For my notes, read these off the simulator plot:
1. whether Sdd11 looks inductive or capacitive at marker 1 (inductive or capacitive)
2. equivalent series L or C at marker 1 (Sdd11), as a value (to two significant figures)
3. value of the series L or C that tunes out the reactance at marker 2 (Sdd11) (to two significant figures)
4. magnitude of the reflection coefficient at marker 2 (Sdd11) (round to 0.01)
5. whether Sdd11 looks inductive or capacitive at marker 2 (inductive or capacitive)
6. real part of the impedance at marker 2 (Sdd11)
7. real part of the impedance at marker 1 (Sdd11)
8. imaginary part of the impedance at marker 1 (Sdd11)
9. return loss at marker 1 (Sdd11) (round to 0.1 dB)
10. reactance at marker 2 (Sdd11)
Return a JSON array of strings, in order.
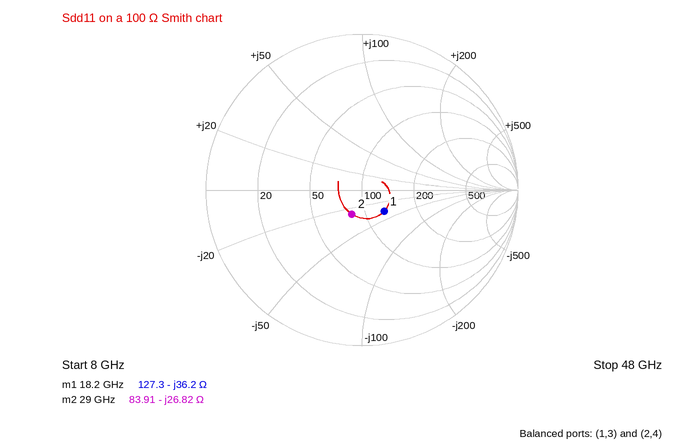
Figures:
["capacitive", "240 fF", "150 pH", "0.17", "capacitive", "83.91 Ω", "127.3 Ω", "-36.2 Ω", "14.1 dB", "-26.82 Ω"]
